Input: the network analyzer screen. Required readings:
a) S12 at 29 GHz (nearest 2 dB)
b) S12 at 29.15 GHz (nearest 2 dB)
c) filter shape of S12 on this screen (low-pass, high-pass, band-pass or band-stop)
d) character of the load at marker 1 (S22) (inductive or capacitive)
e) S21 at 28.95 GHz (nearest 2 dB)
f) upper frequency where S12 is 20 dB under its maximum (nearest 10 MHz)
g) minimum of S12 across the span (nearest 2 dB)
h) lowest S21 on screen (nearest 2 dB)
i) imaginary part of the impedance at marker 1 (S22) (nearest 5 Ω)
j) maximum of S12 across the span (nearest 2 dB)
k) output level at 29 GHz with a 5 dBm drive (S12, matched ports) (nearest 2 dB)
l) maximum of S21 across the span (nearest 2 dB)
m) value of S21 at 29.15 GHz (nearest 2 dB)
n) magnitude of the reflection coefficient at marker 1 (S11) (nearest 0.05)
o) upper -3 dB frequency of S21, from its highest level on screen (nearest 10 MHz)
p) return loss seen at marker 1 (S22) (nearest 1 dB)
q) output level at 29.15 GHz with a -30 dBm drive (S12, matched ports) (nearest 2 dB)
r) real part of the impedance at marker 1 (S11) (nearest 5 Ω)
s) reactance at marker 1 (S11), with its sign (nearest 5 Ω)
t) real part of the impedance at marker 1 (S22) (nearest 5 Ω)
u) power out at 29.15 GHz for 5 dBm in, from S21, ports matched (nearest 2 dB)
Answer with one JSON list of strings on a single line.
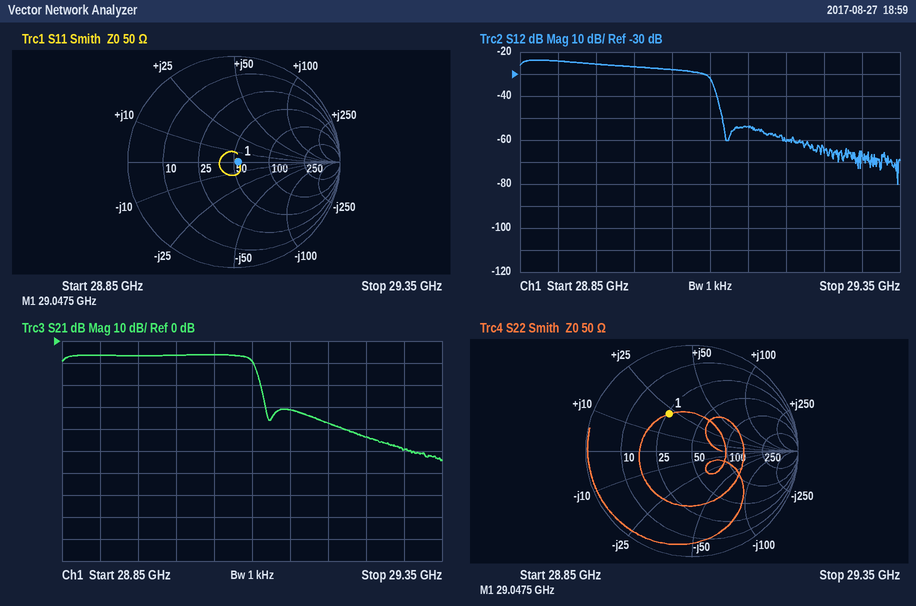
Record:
["-26 dB", "-54 dB", "low-pass", "inductive", "-6 dB", "29.11 GHz", "-80 dB", "-54 dB", "+20 Ω", "-24 dB", "-22 dBm", "-6 dB", "-32 dB", "0.05", "29.10 GHz", "8 dB", "-84 dBm", "55 Ω", "0 Ω", "25 Ω", "-26 dBm"]
